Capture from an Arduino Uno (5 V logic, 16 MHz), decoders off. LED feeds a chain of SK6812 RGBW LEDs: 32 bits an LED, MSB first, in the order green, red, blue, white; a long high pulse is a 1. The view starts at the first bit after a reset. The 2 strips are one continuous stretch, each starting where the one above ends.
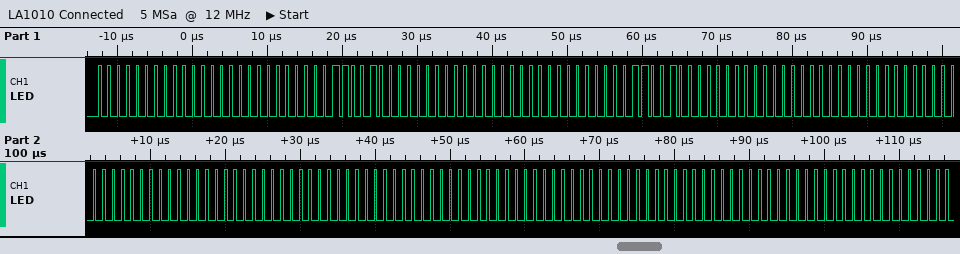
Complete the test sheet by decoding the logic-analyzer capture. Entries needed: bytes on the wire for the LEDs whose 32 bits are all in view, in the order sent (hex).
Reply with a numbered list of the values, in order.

1. 00 00 00 64 00 00 00 64 00 00 00 00 00 00 00 00 00 00 00 00
